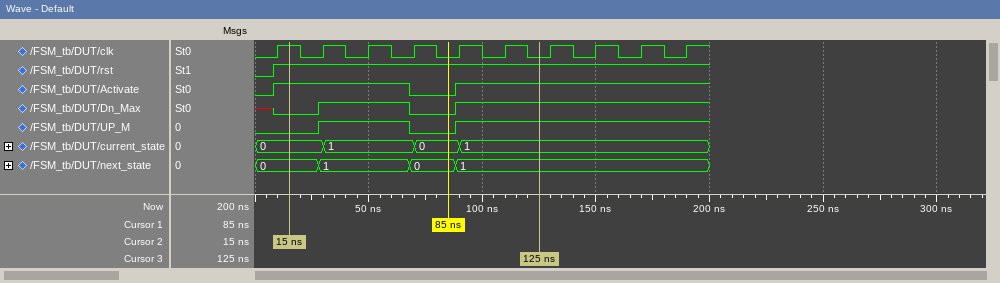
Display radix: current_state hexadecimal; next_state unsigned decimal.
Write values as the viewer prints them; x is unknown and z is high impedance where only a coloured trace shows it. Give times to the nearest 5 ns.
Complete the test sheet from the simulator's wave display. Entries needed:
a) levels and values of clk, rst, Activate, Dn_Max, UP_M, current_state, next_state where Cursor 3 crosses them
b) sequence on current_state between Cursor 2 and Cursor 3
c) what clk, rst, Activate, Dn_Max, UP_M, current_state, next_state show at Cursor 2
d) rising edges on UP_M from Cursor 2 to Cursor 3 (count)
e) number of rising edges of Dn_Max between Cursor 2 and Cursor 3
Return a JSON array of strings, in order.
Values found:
["clk=0, rst=1, Activate=1, Dn_Max=1, UP_M=1, current_state=1, next_state=1", "0, 1, 0, 1", "clk=1, rst=1, Activate=1, Dn_Max=0, UP_M=0, current_state=0, next_state=0", "2", "2"]
